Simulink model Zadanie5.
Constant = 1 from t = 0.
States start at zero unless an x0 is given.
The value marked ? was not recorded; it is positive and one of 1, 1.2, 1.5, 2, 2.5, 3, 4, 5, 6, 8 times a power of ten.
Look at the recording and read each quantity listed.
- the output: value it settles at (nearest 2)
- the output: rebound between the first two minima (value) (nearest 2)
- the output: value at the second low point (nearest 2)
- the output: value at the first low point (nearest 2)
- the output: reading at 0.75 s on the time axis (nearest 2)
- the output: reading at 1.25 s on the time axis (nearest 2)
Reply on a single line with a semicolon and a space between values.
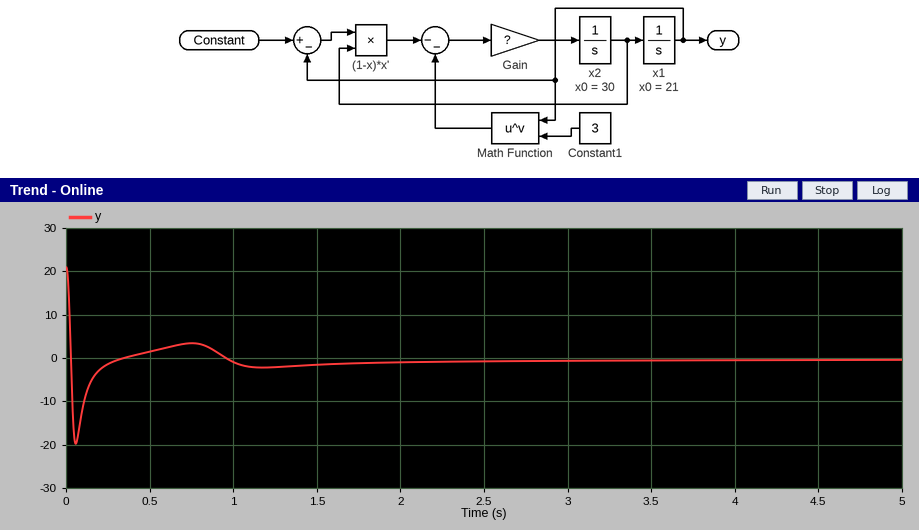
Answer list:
0; 4; -2; -20; 4; -2
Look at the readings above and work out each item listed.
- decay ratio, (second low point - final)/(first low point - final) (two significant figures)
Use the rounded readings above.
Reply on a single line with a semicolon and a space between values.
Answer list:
0.10
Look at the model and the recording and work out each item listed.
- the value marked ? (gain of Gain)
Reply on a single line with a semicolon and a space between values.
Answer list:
4
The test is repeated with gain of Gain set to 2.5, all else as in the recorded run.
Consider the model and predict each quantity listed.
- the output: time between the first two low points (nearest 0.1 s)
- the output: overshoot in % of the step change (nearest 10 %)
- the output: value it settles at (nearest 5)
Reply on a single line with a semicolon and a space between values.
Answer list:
0.4 s; 90 %; 0
